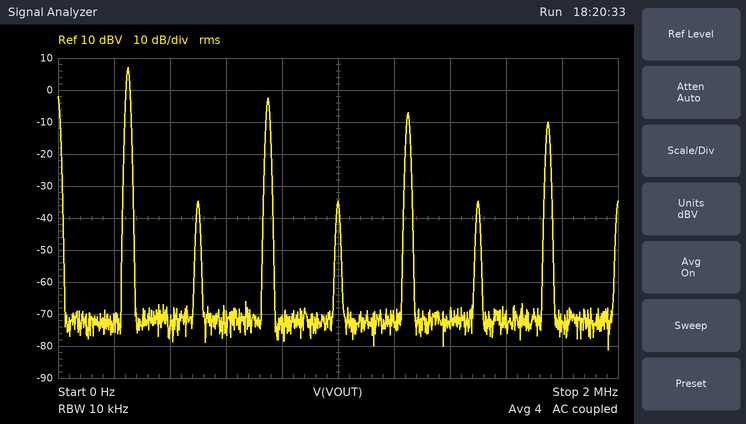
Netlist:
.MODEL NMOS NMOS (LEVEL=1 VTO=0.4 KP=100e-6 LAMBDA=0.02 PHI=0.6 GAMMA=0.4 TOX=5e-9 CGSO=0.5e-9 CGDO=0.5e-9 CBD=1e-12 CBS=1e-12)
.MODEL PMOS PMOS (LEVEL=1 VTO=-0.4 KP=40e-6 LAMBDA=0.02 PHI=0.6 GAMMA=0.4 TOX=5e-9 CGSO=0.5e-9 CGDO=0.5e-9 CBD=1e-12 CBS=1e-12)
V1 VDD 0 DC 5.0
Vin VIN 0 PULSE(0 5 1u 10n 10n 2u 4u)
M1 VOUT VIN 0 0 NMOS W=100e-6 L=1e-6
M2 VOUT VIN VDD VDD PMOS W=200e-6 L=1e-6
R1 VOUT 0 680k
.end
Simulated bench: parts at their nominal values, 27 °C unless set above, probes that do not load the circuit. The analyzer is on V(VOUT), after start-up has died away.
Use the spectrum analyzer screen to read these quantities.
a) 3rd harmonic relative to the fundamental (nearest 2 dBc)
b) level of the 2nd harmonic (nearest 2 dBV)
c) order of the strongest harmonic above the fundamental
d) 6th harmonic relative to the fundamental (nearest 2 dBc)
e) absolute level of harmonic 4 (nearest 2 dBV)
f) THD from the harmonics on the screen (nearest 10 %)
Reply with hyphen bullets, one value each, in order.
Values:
- -10 dBc
- -34 dBV
- 3
- -42 dBc
- -34 dBV
- 40 %
